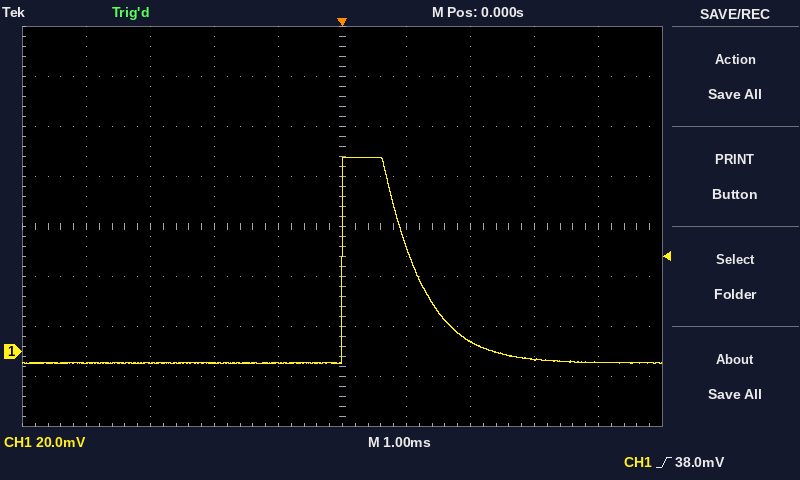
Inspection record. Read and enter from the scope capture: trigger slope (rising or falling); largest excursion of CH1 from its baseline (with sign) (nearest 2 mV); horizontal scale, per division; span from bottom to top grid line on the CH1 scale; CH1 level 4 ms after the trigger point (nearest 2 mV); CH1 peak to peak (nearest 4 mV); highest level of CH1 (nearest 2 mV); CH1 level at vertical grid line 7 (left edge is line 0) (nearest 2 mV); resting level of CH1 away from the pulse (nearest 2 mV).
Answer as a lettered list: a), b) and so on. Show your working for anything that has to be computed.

a) rising
b) 78 mV − (-4 mV) = +82 mV
c) 1 ms
d) 160 mV
e) -4 mV
f) 84 mV
g) 78 mV
h) 4 mV
i) -4 mV
